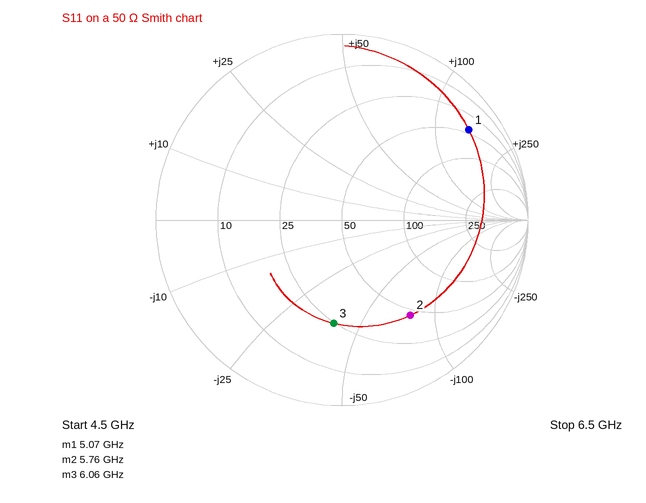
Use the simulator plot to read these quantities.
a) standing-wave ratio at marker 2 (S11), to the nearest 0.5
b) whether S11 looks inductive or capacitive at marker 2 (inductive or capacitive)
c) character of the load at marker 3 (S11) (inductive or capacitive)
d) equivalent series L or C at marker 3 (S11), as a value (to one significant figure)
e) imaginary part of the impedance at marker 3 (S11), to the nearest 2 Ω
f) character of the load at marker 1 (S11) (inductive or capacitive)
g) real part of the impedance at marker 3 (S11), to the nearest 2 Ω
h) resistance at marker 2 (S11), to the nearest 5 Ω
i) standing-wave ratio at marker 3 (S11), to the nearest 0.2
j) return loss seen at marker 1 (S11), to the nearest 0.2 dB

4.5
capacitive
capacitive
700 fF
-40 Ω
inductive
24 Ω
45 Ω
3.6
1.6 dB
